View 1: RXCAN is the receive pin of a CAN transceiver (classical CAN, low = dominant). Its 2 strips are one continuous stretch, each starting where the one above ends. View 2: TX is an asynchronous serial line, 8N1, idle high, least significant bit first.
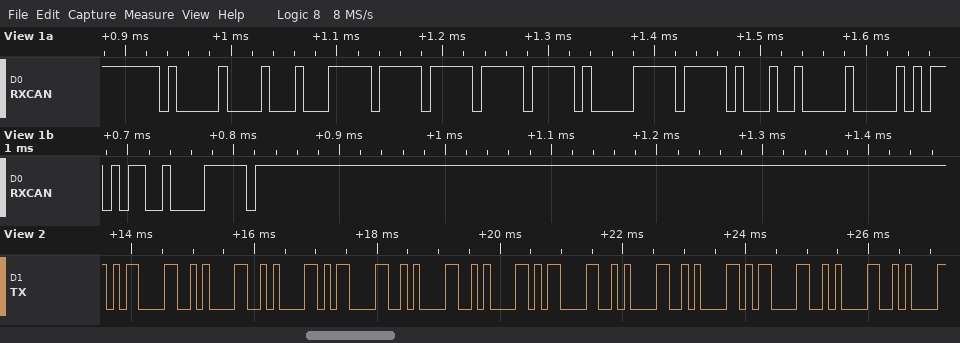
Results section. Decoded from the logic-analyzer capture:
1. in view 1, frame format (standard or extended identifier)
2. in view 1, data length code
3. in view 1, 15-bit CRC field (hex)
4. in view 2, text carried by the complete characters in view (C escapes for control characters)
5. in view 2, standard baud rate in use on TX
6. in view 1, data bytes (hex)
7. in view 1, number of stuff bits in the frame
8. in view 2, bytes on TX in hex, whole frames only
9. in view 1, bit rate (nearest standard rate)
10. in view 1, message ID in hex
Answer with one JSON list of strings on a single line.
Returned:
["standard", "8", "0x590F", "\"\\r\\n\\n\\r\\n\\n\\r\\n\\n\\r\\n\\n\"", "9600 baud", "FF FF FF C1 FF 89 00 16", "11", "0x0D 0x0A 0x0A 0x0D 0x0A 0x0A 0x0D 0x0A 0x0A 0x0D 0x0A 0x0A", "125 kbit/s", "0x401"]
